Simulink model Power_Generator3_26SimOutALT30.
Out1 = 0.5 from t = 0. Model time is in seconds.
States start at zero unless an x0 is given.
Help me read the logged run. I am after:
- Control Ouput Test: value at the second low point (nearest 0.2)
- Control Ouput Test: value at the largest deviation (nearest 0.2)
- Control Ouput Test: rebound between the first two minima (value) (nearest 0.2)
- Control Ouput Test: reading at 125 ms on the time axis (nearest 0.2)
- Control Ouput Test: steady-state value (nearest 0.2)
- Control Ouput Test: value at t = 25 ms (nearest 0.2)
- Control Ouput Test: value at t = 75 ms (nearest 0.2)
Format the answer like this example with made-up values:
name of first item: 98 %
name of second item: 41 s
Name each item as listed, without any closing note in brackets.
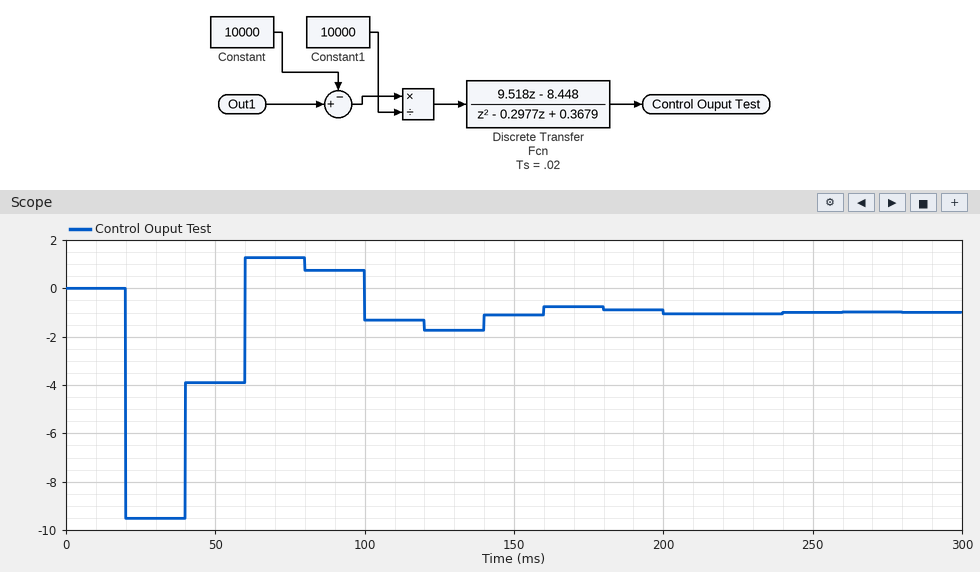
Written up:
Control Ouput Test: value at the second low point: -1.8
Control Ouput Test: value at the largest deviation: -9.6
Control Ouput Test: rebound between the first two minima (value): 1.2
Control Ouput Test: reading at 125 ms on the time axis: -1.8
Control Ouput Test: steady-state value: -1.0
Control Ouput Test: value at t = 25 ms: -9.6
Control Ouput Test: value at t = 75 ms: 1.2
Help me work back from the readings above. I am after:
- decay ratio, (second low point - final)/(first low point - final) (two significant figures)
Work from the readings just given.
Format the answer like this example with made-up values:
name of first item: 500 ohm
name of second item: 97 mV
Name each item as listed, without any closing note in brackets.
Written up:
decay ratio, (second low point - final)/(first low point - final): 0.093
